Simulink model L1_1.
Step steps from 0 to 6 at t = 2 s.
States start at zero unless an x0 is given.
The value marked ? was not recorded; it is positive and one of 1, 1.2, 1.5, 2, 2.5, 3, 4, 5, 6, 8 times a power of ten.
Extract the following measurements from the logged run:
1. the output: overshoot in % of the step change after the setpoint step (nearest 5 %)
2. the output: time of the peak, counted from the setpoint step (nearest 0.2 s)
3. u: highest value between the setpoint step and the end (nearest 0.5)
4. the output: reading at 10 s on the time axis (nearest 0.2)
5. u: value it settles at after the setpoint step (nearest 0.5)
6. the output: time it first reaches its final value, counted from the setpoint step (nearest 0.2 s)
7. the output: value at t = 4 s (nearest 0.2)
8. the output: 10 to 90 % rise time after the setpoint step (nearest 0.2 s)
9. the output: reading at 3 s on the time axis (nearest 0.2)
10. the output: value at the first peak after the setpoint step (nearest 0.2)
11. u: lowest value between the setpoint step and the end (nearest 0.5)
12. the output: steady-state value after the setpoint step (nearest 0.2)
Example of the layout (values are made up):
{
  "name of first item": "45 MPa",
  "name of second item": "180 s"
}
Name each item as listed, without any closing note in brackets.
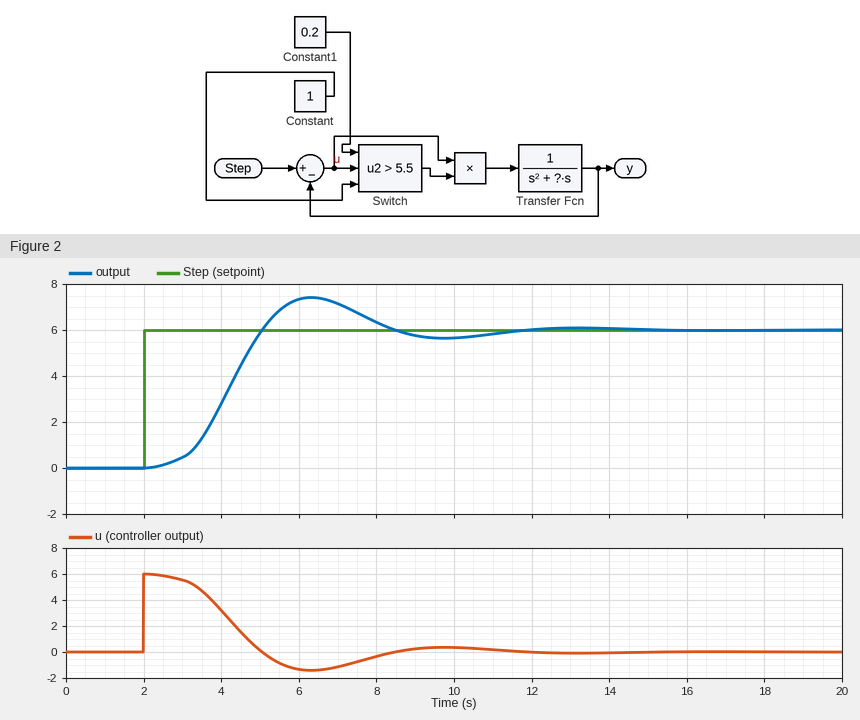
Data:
{
  "the output: overshoot in % of the step change after the setpoint step": "25 %",
  "the output: time of the peak, counted from the setpoint step": "4.4 s",
  "u: highest value between the setpoint step and the end": "6.0",
  "the output: reading at 10 s on the time axis": "5.6",
  "u: value it settles at after the setpoint step": "0.0",
  "the output: time it first reaches its final value, counted from the setpoint step": "3.0 s",
  "the output: value at t = 4 s": "2.8",
  "the output: 10 to 90 % rise time after the setpoint step": "1.6 s",
  "the output: reading at 3 s on the time axis": "0.4",
  "the output: value at the first peak after the setpoint step": "7.4",
  "u: lowest value between the setpoint step and the end": "-1.5",
  "the output: steady-state value after the setpoint step": "6.0"
}
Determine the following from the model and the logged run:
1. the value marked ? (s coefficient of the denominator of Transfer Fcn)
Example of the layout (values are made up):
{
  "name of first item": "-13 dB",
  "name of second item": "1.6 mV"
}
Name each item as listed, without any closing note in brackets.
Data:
{
  "the value marked ?": "0.8"
}
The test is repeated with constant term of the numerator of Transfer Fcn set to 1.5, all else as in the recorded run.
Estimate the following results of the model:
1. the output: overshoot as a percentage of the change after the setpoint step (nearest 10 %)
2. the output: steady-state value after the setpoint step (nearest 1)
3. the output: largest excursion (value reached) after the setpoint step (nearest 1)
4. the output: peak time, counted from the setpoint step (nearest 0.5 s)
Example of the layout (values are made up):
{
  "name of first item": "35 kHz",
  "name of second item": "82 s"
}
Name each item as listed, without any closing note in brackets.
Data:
{
  "the output: overshoot as a percentage of the change after the setpoint step": "30 %",
  "the output: steady-state value after the setpoint step": "6",
  "the output: largest excursion (value reached) after the setpoint step": "8",
  "the output: peak time, counted from the setpoint step": "3.5 s"
}
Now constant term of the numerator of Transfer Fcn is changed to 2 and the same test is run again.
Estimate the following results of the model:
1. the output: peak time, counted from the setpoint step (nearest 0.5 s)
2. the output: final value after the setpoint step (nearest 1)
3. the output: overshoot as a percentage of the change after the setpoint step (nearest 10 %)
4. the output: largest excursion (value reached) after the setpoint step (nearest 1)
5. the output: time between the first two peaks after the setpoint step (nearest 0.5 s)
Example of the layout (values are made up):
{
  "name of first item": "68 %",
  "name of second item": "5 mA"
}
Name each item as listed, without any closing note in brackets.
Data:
{
  "the output: peak time, counted from the setpoint step": "3.0 s",
  "the output: final value after the setpoint step": "6",
  "the output: overshoot as a percentage of the change after the setpoint step": "40 %",
  "the output: largest excursion (value reached) after the setpoint step": "8",
  "the output: time between the first two peaks after the setpoint step": "4.5 s"
}
